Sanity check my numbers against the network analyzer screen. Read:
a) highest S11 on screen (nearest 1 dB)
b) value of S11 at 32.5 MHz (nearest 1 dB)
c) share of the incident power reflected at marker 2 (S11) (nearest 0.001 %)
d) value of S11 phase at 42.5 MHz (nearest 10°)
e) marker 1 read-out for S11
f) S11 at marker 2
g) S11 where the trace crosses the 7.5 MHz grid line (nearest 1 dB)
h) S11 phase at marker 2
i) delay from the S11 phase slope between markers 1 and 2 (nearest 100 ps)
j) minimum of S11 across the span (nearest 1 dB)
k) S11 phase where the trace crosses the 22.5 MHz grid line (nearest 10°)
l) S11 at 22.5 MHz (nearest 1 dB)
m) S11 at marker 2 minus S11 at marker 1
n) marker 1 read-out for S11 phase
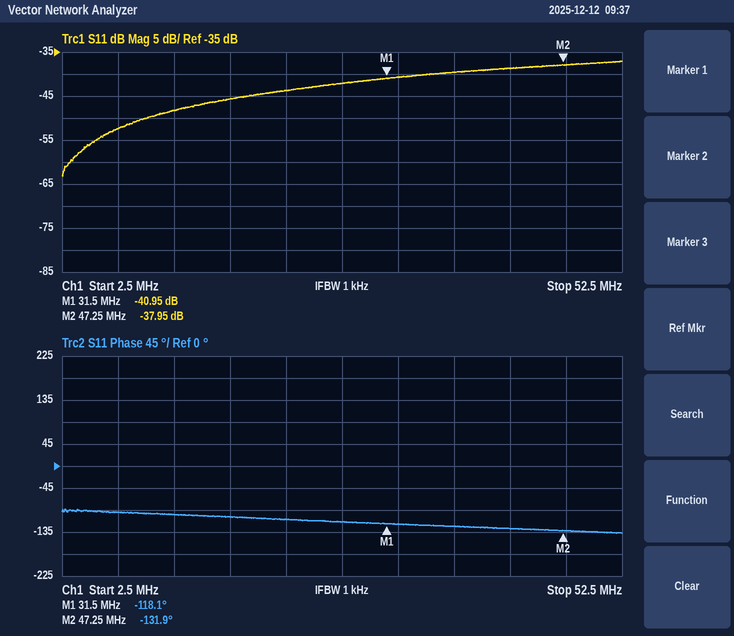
-37 dB
-41 dB
0.016 %
-130°
-40.95 dB
-37.95 dB
-52 dB
-131.9°
2.4 ns
-63 dB
-110°
-44 dB
3.00 dB
-118.1°
